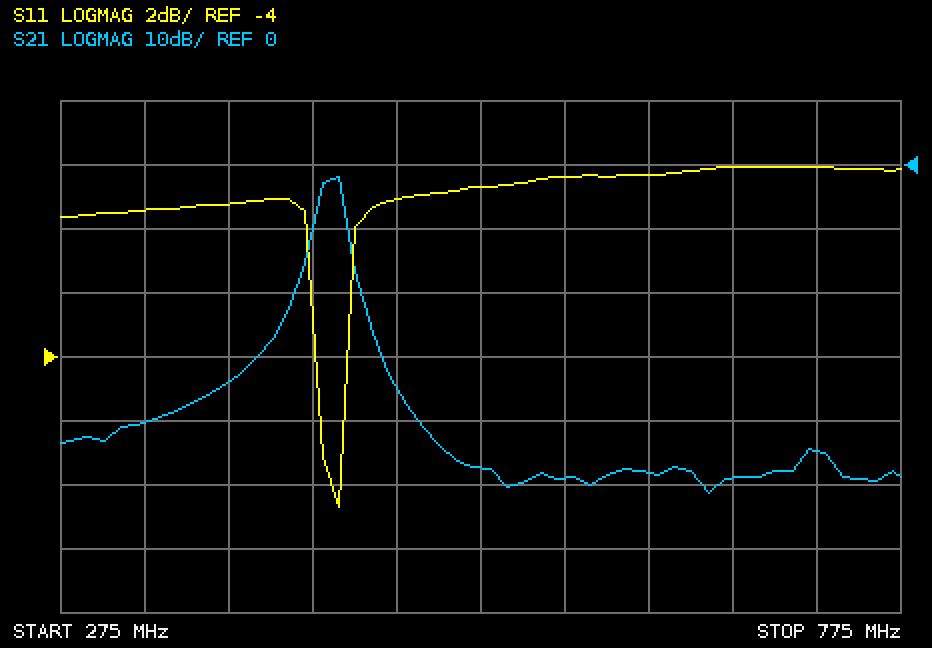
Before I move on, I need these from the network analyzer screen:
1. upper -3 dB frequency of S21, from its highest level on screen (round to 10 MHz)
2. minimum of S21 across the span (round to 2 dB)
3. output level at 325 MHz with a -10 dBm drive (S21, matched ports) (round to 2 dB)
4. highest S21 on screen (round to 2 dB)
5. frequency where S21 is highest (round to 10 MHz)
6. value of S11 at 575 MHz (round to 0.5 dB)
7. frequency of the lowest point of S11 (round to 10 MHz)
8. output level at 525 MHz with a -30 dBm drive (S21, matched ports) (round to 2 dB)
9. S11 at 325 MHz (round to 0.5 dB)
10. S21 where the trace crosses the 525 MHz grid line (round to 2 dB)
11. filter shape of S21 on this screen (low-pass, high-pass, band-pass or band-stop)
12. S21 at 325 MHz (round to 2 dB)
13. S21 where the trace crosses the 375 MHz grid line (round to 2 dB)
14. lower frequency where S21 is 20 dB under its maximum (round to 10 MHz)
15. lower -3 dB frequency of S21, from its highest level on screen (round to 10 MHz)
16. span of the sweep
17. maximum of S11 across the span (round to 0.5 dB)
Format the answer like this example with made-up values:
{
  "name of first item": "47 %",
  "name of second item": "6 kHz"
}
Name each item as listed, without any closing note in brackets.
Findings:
{
  "upper -3 dB frequency of S21, from its highest level on screen": "440 MHz",
  "minimum of S21 across the span": "-52 dB",
  "output level at 325 MHz with a -10 dBm drive (S21, matched ports)": "-50 dBm",
  "highest S21 on screen": "-2 dB",
  "frequency where S21 is highest": "440 MHz",
  "value of S11 at 575 MHz": "1.5 dB",
  "frequency of the lowest point of S11": "440 MHz",
  "output level at 525 MHz with a -30 dBm drive (S21, matched ports)": "-78 dBm",
  "S11 at 325 MHz": "0.5 dB",
  "S21 where the trace crosses the 525 MHz grid line": "-48 dB",
  "filter shape of S21 on this screen": "band-pass",
  "S21 at 325 MHz": "-40 dB",
  "S21 where the trace crosses the 375 MHz grid line": "-34 dB",
  "lower frequency where S21 is 20 dB under its maximum": "410 MHz",
  "lower -3 dB frequency of S21, from its highest level on screen": "430 MHz",
  "span of the sweep": "500 MHz",
  "maximum of S11 across the span": "2.0 dB"
}
